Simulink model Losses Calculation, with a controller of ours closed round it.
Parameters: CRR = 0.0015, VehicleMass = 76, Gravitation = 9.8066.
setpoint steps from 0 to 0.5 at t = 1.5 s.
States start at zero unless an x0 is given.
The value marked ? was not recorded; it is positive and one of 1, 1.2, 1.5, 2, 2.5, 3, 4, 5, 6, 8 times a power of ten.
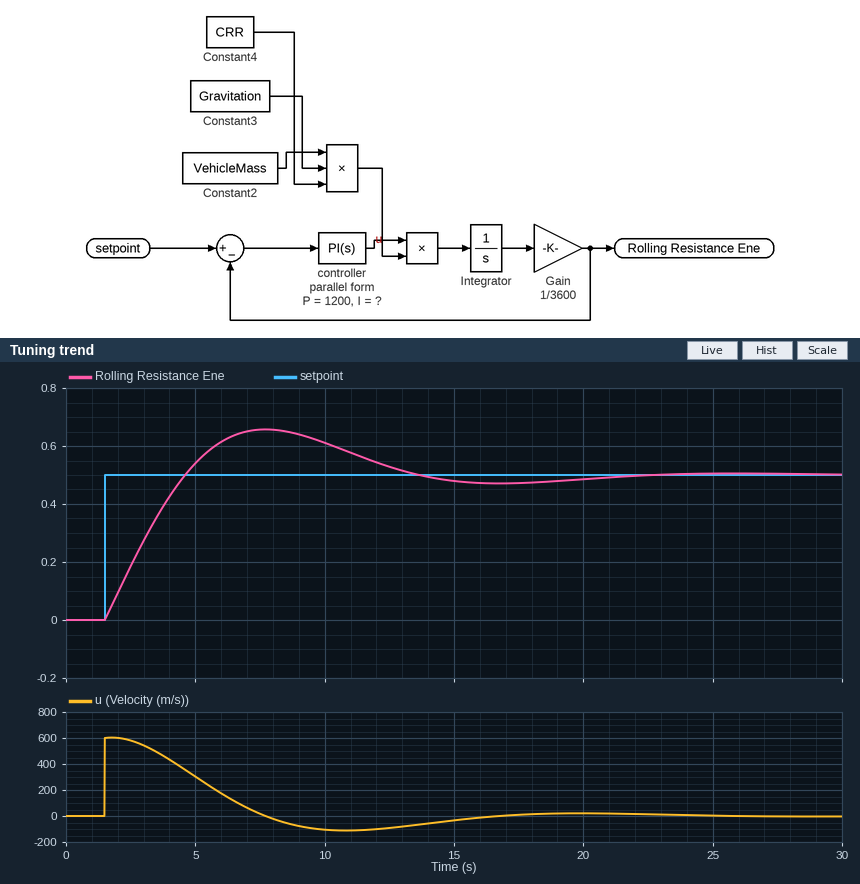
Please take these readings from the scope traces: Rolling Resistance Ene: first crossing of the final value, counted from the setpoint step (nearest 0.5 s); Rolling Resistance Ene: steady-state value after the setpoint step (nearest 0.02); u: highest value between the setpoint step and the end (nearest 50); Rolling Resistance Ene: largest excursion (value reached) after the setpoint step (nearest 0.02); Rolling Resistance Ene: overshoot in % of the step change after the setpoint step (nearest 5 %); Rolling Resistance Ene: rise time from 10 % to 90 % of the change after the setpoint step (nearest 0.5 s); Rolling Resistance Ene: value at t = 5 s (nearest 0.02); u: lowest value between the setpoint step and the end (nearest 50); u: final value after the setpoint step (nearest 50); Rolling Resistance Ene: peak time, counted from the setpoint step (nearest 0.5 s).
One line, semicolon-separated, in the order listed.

3.0 s; 0.50; 600; 0.66; 30 %; 2.5 s; 0.54; -100; 0; 6.0 s
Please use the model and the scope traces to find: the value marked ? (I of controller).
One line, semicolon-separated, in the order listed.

500
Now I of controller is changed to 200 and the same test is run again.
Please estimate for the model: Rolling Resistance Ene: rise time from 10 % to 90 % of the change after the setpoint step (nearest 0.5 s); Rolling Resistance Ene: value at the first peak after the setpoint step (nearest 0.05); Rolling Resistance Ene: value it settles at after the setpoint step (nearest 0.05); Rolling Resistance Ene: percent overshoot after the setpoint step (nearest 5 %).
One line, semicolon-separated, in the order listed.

3.5 s; 0.60; 0.50; 20 %
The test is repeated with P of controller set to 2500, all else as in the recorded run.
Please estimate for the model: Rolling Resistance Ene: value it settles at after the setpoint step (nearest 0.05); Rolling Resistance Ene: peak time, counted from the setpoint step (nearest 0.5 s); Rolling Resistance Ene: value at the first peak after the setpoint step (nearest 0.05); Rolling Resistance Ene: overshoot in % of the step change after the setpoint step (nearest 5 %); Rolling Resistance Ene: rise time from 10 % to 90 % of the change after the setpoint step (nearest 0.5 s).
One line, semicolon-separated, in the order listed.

0.50; 5.0 s; 0.55; 15 %; 2.0 s
